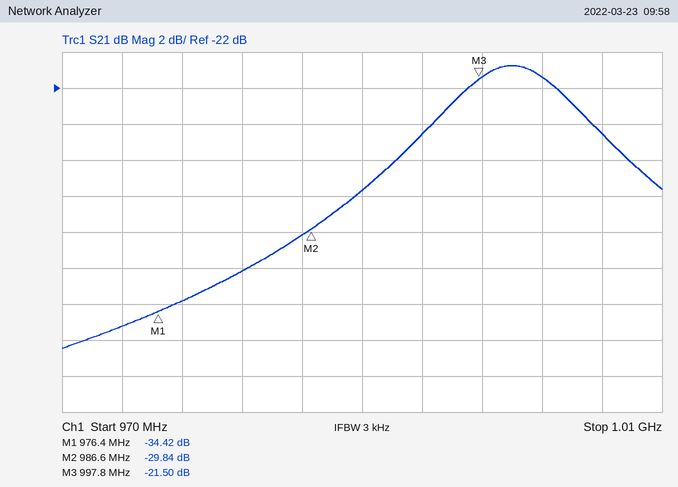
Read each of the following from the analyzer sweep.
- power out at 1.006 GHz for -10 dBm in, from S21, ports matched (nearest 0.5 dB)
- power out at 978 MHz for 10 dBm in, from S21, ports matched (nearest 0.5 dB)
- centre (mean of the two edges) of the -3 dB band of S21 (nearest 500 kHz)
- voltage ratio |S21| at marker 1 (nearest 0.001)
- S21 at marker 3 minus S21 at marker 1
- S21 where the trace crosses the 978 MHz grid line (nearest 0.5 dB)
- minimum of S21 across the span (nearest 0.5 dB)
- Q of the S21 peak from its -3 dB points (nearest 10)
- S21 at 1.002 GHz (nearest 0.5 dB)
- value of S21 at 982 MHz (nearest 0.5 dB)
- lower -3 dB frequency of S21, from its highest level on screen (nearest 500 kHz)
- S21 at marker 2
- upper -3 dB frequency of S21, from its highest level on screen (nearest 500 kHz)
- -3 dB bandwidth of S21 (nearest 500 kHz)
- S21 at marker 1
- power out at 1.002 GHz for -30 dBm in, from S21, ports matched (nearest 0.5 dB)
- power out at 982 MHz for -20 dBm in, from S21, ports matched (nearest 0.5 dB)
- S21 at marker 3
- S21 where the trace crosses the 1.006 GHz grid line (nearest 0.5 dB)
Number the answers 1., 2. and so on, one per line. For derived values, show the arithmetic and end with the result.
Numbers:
1. -10 dBm + (-24.5 dB) = -34.5 dBm
2. 10 dBm + (-34.0 dB) = -24.0 dBm
3. 1.0000 GHz
4. 10^(-34.42/20) ≈ 0.019
5. -21.5 − (-34.42) = 12.92 dB
6. -34.0 dB
7. -36.5 dB
8. 1 GHz / 10 MHz ≈ 100
9. -21.5 dB
10. -32.0 dB
11. 995.0 MHz
12. -29.84 dB
13. 1.0050 GHz
14. 1.0050 GHz − 995.0 MHz = 10.0 MHz
15. -34.42 dB
16. -30 dBm + (-21.5 dB) = -51.5 dBm
17. -20 dBm + (-32.0 dB) = -52.0 dBm
18. -21.50 dB
19. -24.5 dB
